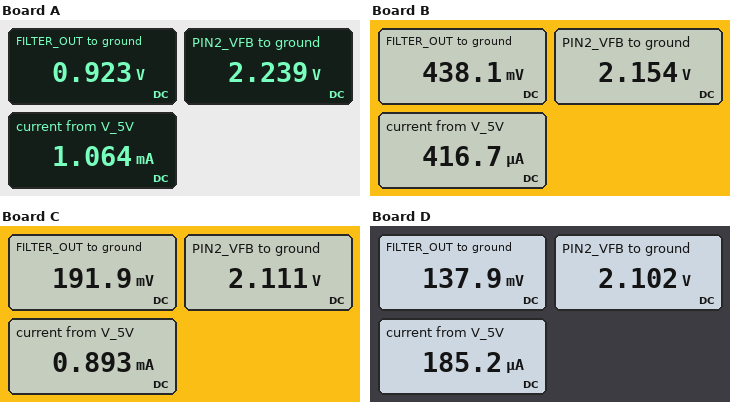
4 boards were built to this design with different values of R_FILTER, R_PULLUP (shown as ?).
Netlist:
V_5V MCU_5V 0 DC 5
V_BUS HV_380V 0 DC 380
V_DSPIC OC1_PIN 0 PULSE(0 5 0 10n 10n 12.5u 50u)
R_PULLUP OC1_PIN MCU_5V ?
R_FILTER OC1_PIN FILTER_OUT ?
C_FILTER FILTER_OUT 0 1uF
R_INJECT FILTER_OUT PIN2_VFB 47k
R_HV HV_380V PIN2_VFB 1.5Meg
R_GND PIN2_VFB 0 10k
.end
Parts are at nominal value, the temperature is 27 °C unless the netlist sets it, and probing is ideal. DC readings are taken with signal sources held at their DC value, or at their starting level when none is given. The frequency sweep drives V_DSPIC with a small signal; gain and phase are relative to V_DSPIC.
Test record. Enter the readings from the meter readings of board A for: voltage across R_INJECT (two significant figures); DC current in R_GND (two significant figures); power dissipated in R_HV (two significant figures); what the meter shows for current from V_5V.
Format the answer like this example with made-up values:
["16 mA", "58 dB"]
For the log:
["1.3 V", "220 µA", "95 mW", "1.064 mA"]
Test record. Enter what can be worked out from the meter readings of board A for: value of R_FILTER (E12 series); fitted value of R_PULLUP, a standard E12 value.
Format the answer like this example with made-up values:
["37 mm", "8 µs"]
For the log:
["33 kΩ", "4.7 kΩ"]
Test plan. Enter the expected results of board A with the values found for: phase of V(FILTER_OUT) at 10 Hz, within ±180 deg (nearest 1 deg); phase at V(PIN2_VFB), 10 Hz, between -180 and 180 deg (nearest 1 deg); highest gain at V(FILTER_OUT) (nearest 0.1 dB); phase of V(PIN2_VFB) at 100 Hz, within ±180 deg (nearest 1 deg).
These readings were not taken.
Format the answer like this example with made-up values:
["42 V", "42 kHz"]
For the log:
["-53 deg", "-53 deg", "-4.0 dB", "-86 deg"]
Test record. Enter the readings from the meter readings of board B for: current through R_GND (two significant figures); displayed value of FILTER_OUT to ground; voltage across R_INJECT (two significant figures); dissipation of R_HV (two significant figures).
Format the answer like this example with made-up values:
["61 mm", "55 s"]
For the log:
["220 µA", "438.1 mV", "1.7 V", "95 mW"]
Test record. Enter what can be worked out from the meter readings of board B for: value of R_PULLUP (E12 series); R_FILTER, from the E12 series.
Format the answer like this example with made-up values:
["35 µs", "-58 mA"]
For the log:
["12 kΩ", "12 kΩ"]
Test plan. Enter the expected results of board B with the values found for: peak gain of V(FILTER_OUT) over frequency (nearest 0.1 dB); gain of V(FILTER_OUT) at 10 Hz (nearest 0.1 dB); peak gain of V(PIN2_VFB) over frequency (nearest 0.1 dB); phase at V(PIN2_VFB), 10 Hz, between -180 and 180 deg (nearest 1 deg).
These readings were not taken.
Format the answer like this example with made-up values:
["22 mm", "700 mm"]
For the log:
["-1.7 dB", "-3.1 dB", "-16.8 dB", "-32 deg"]
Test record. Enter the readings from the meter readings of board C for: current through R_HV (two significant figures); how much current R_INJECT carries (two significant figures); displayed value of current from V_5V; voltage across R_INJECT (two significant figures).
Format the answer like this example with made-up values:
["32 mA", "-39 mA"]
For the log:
["250 µA", "41 µA", "0.893 mA", "1.9 V"]
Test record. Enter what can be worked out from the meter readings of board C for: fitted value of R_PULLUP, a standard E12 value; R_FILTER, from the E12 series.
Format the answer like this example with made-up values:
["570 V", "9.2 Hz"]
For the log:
["5.6 kΩ", "4.7 kΩ"]
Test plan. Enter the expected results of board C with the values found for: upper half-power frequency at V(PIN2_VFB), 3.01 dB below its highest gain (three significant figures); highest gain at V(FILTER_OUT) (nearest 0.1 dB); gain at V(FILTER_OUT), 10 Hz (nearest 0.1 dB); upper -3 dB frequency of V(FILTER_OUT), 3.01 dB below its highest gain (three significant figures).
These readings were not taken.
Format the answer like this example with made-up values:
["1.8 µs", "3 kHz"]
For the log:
["36.7 Hz", "-0.7 dB", "-1.0 dB", "36.7 Hz"]
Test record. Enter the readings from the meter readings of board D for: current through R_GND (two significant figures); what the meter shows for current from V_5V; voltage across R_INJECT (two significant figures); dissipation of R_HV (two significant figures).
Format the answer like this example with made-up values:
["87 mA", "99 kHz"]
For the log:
["210 µA", "185.2 µA", "2.0 V", "95 mW"]
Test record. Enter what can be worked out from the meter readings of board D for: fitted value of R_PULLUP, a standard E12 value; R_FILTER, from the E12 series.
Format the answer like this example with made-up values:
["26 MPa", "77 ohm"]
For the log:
["27 kΩ", "3.3 kΩ"]
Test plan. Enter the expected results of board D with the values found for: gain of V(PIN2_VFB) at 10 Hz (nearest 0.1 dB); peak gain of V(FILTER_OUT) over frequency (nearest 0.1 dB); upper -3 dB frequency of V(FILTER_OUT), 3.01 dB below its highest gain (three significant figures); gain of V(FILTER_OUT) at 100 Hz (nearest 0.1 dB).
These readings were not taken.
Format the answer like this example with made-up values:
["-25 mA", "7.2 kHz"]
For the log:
["-15.8 dB", "-0.5 dB", "51.0 Hz", "-7.3 dB"]
